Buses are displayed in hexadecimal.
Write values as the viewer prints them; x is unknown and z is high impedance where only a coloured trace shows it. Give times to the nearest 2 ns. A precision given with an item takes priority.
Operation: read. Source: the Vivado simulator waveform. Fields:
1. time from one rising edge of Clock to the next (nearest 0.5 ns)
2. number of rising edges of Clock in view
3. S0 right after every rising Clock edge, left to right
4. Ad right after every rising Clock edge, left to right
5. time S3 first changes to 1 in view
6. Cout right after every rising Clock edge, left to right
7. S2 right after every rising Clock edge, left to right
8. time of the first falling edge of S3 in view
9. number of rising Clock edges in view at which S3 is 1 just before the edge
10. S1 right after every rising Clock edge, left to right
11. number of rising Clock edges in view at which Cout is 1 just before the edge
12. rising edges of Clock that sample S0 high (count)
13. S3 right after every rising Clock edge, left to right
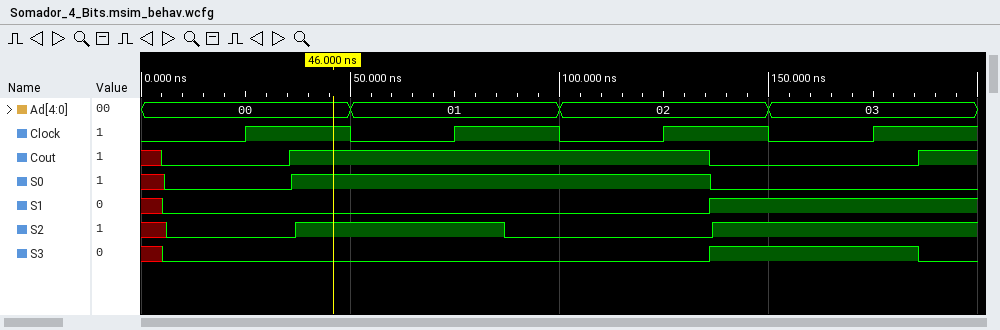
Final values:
50 ns
4
0 1 1 0
00, 01, 02, 03
136 ns
0 1 1 0
0 1 0 1
186 ns
1
0 0 0 1
2
2
0 0 0 1
